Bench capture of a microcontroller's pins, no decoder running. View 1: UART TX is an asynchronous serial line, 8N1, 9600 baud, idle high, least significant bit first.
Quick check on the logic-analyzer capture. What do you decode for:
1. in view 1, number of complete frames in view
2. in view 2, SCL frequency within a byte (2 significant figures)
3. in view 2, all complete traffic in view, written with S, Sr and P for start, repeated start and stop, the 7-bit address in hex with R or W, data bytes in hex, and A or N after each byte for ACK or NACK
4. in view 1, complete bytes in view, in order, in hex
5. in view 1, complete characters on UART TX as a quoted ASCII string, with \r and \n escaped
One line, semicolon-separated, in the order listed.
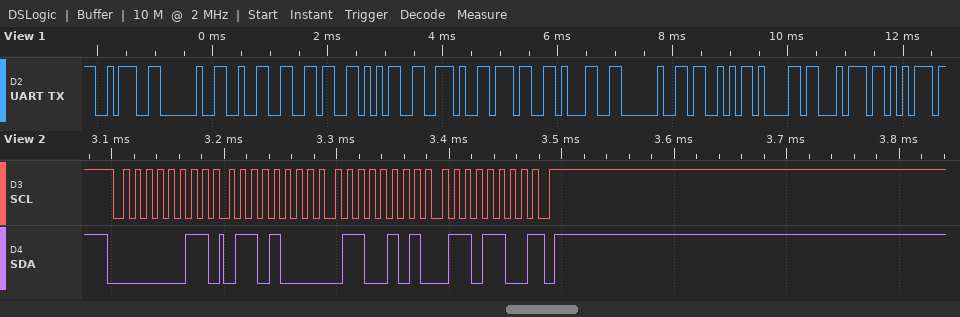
13; 100 kHz; S 01R A 68 A 65 A 6C N P; 0x3A 0x20 0x32 0x36 0x35 0x2E 0x37 0x31 0x20 0x53 0x61 0x74 0x75; ": 265.71 Satu"
